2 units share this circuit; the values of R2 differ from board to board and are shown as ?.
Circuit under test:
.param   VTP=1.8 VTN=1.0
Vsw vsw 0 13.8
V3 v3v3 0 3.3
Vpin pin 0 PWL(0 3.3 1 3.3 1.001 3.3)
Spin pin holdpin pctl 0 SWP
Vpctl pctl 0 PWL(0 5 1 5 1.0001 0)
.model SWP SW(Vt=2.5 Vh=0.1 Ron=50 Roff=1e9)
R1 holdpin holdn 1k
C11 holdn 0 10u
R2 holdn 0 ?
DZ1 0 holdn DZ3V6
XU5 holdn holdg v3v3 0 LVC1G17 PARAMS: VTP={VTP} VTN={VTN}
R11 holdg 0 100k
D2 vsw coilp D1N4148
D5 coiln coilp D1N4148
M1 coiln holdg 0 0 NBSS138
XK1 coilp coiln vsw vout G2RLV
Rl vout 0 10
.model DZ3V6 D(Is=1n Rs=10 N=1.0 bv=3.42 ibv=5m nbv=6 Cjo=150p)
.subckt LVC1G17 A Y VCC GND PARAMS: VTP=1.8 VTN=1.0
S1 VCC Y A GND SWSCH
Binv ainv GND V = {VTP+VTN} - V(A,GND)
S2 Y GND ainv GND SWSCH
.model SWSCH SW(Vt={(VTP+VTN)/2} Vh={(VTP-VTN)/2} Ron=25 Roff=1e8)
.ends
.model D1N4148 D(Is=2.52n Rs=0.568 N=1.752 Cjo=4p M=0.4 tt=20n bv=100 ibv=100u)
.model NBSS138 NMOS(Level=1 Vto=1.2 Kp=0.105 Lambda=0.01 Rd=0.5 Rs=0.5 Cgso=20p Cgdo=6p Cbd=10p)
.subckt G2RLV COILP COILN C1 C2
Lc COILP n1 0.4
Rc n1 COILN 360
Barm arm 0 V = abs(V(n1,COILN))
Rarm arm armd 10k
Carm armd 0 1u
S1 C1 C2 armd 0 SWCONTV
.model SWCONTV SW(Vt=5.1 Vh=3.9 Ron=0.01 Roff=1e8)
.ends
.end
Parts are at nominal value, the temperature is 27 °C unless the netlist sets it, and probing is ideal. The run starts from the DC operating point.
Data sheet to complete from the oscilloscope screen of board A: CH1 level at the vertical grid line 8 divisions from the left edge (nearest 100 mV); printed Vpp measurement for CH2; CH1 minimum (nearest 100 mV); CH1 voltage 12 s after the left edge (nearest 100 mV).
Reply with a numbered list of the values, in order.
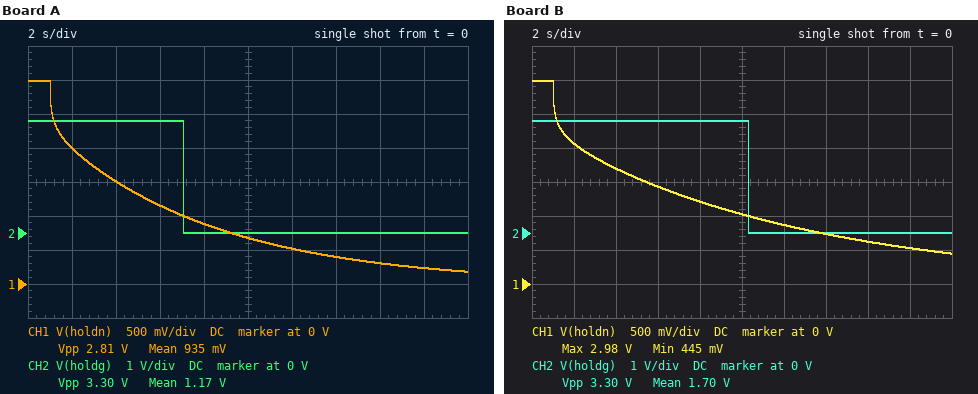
1. 300 mV
2. 3.30 V
3. 200 mV
4. 500 mV
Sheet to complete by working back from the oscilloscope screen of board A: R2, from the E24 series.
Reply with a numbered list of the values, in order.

1. 750 kΩ
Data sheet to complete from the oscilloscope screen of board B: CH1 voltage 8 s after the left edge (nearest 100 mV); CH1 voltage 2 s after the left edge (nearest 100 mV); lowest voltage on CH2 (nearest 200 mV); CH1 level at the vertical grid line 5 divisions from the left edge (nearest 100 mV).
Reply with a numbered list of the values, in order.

1. 1.2 V
2. 2.1 V
3. 0 V
4. 1.0 V
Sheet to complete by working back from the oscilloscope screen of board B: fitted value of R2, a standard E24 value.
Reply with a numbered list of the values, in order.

1. 1.2 MΩ
